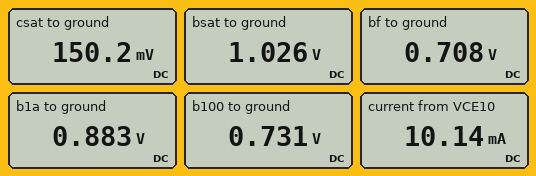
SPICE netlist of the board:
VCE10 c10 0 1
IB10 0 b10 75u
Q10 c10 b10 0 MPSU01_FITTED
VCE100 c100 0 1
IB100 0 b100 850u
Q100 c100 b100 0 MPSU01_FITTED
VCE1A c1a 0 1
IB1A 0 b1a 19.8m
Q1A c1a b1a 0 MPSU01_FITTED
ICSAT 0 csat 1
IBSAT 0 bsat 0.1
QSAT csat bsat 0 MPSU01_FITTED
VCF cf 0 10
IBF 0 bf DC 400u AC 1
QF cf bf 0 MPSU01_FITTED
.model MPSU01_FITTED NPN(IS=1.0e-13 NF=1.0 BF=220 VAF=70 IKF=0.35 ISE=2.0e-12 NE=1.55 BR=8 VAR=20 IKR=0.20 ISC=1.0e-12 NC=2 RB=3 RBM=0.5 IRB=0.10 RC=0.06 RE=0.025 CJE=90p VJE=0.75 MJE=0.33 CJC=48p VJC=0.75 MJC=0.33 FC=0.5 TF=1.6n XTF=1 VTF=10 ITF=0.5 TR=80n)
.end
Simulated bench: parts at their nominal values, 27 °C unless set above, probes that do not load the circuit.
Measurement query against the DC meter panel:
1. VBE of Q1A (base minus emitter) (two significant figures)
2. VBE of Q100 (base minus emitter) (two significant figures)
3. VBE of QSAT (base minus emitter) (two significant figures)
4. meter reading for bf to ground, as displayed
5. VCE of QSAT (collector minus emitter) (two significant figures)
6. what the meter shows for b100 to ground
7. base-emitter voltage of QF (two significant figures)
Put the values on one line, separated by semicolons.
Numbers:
880 mV; 730 mV; 1.0 V; 0.708 V; 150 mV; 0.731 V; 710 mV
